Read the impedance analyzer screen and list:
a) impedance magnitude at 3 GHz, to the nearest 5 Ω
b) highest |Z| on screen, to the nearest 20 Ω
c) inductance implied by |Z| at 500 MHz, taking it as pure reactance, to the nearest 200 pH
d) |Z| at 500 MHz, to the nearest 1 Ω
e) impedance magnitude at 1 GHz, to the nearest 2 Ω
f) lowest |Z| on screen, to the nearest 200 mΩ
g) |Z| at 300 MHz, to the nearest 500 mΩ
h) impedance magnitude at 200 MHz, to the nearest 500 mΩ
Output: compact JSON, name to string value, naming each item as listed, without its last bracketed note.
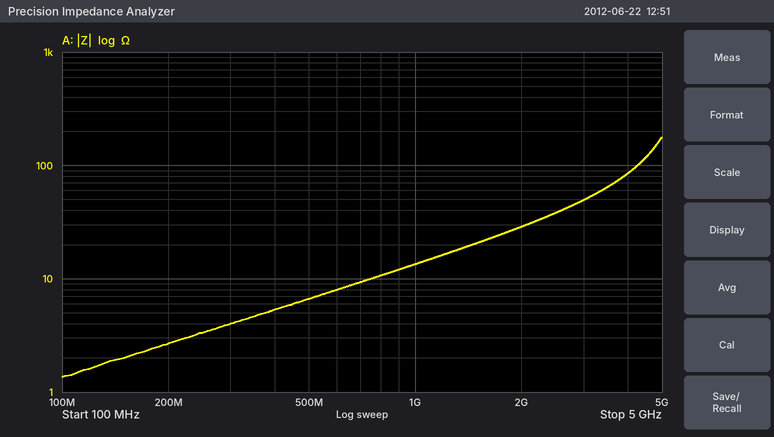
{"impedance magnitude at 3 GHz, to the nearest 5 Ω": "50 Ω", "highest |Z| on screen, to the nearest 20 Ω": "180 Ω", "inductance implied by |Z| at 500 MHz, taking it as pure reactance, to the nearest 200 pH": "2.2 nH", "|Z| at 500 MHz, to the nearest 1 Ω": "7 Ω", "impedance magnitude at 1 GHz, to the nearest 2 Ω": "14 Ω", "lowest |Z| on screen, to the nearest 200 mΩ": "1.4 Ω", "|Z| at 300 MHz, to the nearest 500 mΩ": "4.0 Ω", "impedance magnitude at 200 MHz, to the nearest 500 mΩ": "2.5 Ω"}
